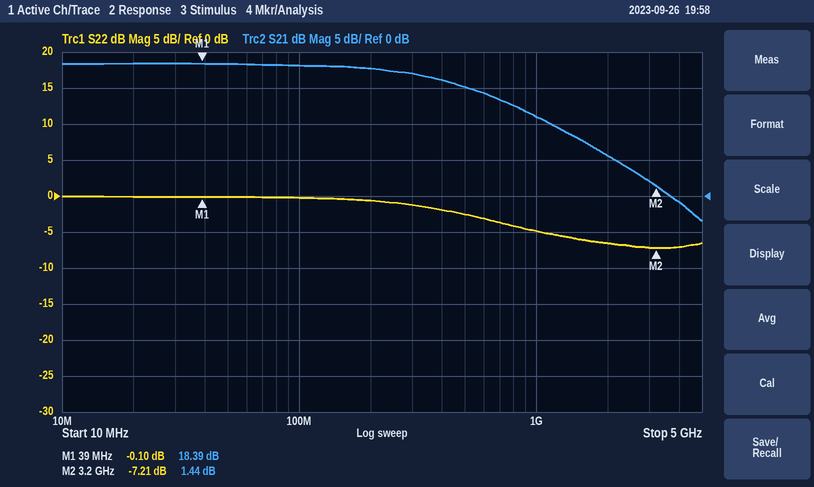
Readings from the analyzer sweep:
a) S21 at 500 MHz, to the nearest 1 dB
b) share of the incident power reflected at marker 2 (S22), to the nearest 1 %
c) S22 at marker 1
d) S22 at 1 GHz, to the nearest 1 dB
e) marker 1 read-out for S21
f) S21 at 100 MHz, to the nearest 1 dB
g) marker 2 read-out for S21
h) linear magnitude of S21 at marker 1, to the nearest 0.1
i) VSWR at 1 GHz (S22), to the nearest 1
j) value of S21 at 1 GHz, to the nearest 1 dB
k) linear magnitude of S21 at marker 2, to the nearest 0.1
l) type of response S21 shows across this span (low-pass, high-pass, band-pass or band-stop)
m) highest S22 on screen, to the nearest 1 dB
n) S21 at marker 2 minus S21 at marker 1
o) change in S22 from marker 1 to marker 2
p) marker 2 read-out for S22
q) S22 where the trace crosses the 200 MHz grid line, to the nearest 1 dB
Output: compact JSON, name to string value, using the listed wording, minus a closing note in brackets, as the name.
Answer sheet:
{"S21 at 500 MHz, to the nearest 1 dB": "15 dB", "share of the incident power reflected at marker 2 (S22), to the nearest 1 %": "19 %", "S22 at marker 1": "-0.10 dB", "S22 at 1 GHz, to the nearest 1 dB": "-5 dB", "marker 1 read-out for S21": "18.39 dB", "S21 at 100 MHz, to the nearest 1 dB": "18 dB", "marker 2 read-out for S21": "1.44 dB", "linear magnitude of S21 at marker 1, to the nearest 0.1": "8.3", "VSWR at 1 GHz (S22), to the nearest 1": "4", "value of S21 at 1 GHz, to the nearest 1 dB": "11 dB", "linear magnitude of S21 at marker 2, to the nearest 0.1": "1.2", "type of response S21 shows across this span": "low-pass", "highest S22 on screen, to the nearest 1 dB": "0 dB", "S21 at marker 2 minus S21 at marker 1": "-16.95 dB", "change in S22 from marker 1 to marker 2": "-7.11 dB", "marker 2 read-out for S22": "-7.21 dB", "S22 where the trace crosses the 200 MHz grid line, to the nearest 1 dB": "-1 dB"}
